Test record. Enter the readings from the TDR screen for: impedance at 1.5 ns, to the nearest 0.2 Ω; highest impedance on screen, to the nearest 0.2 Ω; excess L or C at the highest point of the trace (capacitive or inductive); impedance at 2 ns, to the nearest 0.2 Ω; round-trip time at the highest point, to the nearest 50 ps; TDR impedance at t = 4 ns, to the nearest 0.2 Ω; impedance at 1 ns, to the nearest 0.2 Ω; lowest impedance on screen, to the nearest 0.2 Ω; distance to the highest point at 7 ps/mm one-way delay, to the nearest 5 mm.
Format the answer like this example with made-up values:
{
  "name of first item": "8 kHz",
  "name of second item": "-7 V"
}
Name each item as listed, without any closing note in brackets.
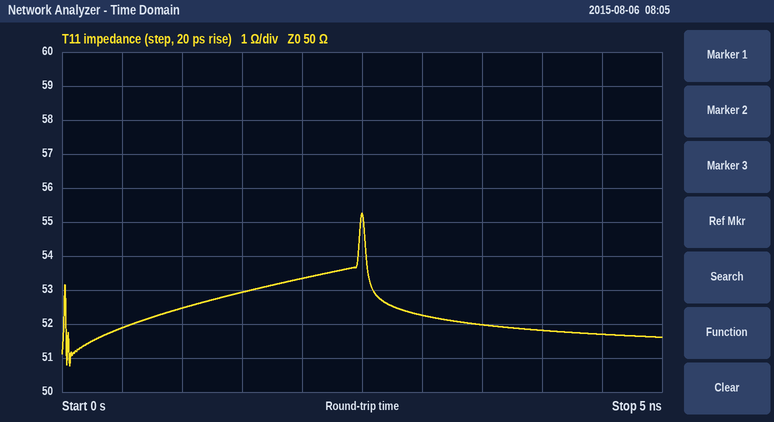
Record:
{
  "impedance at 1.5 ns, to the nearest 0.2 Ω": "53.0 Ω",
  "highest impedance on screen, to the nearest 0.2 Ω": "55.2 Ω",
  "excess L or C at the highest point of the trace": "inductive",
  "impedance at 2 ns, to the nearest 0.2 Ω": "53.4 Ω",
  "round-trip time at the highest point, to the nearest 50 ps": "2.50 ns",
  "TDR impedance at t = 4 ns, to the nearest 0.2 Ω": "51.8 Ω",
  "impedance at 1 ns, to the nearest 0.2 Ω": "52.4 Ω",
  "lowest impedance on screen, to the nearest 0.2 Ω": "50.8 Ω",
  "distance to the highest point at 7 ps/mm one-way delay, to the nearest 5 mm": "180 mm"
}
